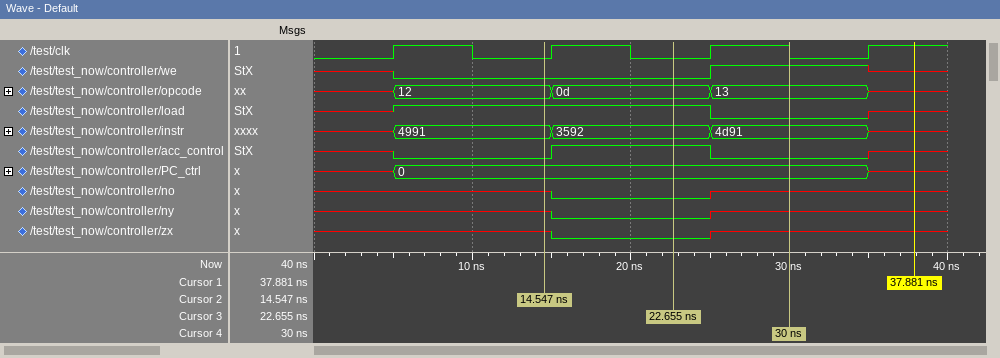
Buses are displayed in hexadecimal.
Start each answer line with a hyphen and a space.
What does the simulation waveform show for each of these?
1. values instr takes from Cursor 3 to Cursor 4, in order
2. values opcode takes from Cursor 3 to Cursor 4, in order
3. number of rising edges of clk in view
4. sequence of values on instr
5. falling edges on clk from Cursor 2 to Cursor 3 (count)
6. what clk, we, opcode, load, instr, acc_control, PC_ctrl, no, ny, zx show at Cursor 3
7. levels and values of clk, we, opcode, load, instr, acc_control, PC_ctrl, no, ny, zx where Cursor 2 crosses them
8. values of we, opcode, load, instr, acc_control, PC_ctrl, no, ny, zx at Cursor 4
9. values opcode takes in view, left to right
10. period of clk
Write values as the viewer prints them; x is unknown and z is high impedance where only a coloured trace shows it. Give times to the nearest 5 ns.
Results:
- 3592, 4d91
- 0d, 13
- 4
- x, 4991, 3592, 4d91, x
- 1
- clk=0, we=0, opcode=0d, load=1, instr=3592, acc_control=1, PC_ctrl=0, no=0, ny=0, zx=0
- clk=0, we=0, opcode=12, load=1, instr=4991, acc_control=0, PC_ctrl=0, no=x, ny=x, zx=x
- we=1, opcode=13, load=0, instr=4d91, acc_control=0, PC_ctrl=0, no=x, ny=x, zx=x
- x, 12, 0d, 13, x
- 10 ns
